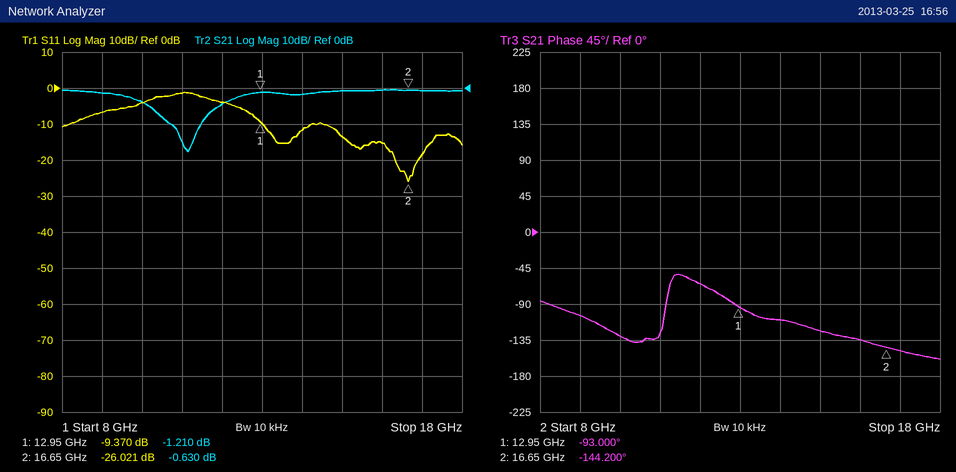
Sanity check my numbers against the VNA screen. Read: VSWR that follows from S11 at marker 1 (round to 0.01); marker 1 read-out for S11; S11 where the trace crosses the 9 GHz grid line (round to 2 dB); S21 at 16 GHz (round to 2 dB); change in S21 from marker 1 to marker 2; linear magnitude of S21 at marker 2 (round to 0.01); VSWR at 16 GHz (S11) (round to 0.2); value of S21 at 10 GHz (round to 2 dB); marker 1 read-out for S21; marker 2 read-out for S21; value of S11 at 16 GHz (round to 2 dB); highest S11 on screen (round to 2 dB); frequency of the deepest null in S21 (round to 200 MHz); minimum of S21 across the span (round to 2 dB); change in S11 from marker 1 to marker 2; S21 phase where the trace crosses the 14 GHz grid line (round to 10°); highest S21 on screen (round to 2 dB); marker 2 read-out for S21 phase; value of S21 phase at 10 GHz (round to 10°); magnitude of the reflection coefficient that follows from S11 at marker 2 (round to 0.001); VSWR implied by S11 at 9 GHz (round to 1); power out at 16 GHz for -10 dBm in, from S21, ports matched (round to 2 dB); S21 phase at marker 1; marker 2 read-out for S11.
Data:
2.03
-9.370 dB
-6 dB
0 dB
0.580 dB
0.93
1.4
-4 dB
-1.210 dB
-0.630 dB
-16 dB
-2 dB
11.2 GHz
-18 dB
-16.651 dB
-110°
0 dB
-144.200°
-130°
0.050
3
-10 dBm
-93.000°
-26.021 dB
